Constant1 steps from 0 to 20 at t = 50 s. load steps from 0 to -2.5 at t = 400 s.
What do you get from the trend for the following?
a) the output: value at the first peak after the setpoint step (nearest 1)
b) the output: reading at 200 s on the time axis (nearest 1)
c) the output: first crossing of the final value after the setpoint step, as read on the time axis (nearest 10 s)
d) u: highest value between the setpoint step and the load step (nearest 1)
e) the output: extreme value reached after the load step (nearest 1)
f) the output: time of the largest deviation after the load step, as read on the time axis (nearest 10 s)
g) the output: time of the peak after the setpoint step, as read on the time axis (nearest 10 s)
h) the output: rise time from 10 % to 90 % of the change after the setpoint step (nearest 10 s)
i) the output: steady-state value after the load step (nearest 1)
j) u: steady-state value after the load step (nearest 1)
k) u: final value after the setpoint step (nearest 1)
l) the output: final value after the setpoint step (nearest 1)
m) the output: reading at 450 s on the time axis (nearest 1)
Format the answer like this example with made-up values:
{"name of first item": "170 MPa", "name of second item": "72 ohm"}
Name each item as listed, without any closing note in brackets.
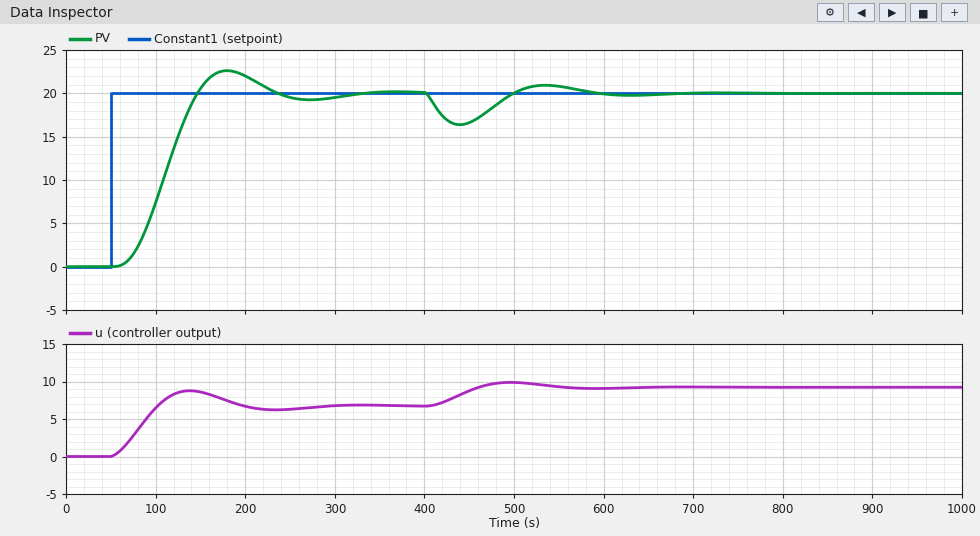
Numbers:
{"the output: value at the first peak after the setpoint step": "23", "the output: reading at 200 s on the time axis": "22", "the output: first crossing of the final value after the setpoint step, as read on the time axis": "150 s", "u: highest value between the setpoint step and the load step": "9", "the output: extreme value reached after the load step": "16", "the output: time of the largest deviation after the load step, as read on the time axis": "440 s", "the output: time of the peak after the setpoint step, as read on the time axis": "180 s", "the output: rise time from 10 % to 90 % of the change after the setpoint step": "60 s", "the output: steady-state value after the load step": "20", "u: steady-state value after the load step": "9", "u: final value after the setpoint step": "7", "the output: final value after the setpoint step": "20", "the output: reading at 450 s on the time axis": "17"}
